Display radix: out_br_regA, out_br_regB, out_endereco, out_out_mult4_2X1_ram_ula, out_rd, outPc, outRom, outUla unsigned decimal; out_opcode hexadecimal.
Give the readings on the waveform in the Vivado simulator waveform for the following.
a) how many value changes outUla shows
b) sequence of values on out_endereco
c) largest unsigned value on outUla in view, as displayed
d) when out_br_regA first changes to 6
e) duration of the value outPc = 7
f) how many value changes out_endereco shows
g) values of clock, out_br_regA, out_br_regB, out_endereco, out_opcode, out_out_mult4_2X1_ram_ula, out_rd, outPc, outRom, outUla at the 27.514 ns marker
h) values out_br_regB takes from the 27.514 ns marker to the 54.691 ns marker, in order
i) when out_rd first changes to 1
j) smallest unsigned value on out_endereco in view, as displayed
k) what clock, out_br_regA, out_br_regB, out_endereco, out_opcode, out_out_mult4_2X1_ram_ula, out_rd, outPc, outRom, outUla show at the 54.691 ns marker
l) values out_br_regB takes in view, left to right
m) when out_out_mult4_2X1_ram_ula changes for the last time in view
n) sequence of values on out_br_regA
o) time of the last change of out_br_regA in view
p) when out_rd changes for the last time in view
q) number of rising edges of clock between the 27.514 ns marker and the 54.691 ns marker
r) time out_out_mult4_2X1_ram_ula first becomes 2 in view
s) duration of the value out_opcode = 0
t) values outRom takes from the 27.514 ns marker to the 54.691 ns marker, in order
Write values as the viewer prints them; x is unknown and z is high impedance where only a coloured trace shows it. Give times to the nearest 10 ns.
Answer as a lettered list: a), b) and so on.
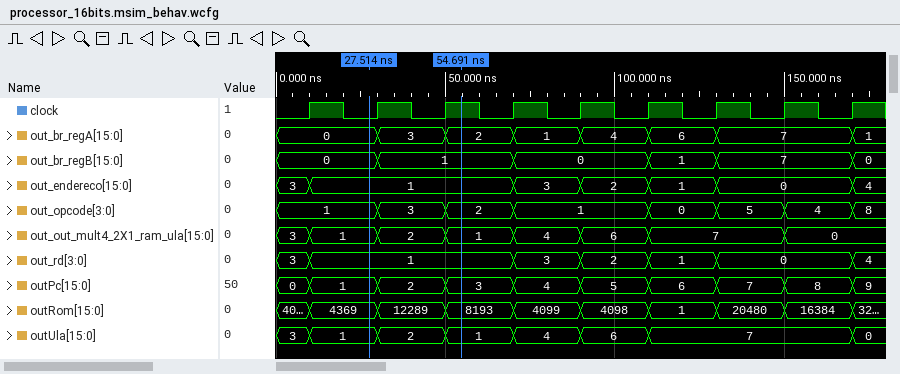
a) 7
b) 3, 1, 3, 2, 1, 0, 4
c) 7
d) 110 ns
e) 20 ns
f) 6
g) clock=0, out_br_regA=0, out_br_regB=0, out_endereco=1, out_opcode=1, out_out_mult4_2X1_ram_ula=1, out_rd=1, outPc=1, outRom=4369, outUla=1
h) 0, 1
i) 10 ns
j) 0
k) clock=1, out_br_regA=2, out_br_regB=1, out_endereco=1, out_opcode=2, out_out_mult4_2X1_ram_ula=1, out_rd=1, outPc=3, outRom=8193, outUla=1
l) 0, 1, 0, 1, 7, 0
m) 150 ns
n) 0, 3, 2, 1, 4, 6, 7, 1
o) 170 ns
p) 170 ns
q) 2
r) 30 ns
s) 20 ns
t) 4369, 12289, 8193
